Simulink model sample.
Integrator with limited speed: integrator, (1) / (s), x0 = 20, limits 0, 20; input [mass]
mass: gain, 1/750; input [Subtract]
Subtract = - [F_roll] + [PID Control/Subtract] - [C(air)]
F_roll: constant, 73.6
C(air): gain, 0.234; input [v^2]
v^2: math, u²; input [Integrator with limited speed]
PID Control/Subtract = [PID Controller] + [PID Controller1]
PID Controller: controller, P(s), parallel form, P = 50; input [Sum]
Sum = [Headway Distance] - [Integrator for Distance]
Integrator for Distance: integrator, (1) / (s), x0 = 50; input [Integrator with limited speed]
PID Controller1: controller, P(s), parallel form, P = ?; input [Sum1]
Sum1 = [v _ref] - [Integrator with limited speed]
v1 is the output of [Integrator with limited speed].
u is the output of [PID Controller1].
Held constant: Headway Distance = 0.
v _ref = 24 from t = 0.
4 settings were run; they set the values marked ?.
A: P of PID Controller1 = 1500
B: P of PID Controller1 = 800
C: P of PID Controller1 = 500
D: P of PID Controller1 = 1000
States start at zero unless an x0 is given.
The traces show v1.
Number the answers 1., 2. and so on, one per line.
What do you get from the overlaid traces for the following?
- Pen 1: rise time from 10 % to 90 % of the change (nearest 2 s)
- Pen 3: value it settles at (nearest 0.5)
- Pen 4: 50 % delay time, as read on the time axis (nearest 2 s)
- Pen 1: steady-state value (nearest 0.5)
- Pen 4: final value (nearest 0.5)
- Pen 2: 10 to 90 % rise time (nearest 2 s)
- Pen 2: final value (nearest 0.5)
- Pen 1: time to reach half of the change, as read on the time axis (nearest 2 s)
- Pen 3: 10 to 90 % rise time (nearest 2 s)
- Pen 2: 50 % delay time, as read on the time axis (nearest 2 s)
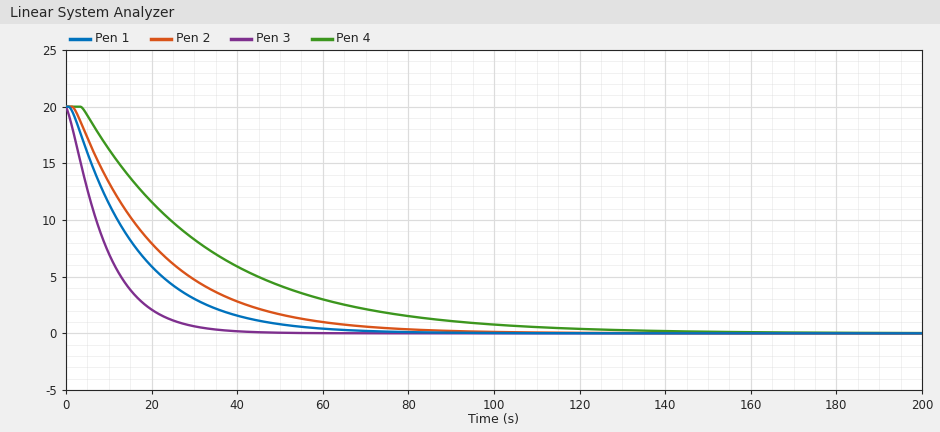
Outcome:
1. 34 s
2. 0.0
3. 24 s
4. 0.0
5. 0.0
6. 42 s
7. 0.0
8. 12 s
9. 18 s
10. 16 s
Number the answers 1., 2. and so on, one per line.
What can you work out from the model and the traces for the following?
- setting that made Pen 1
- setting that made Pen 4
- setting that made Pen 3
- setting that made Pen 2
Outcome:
1. B
2. A
3. C
4. D
